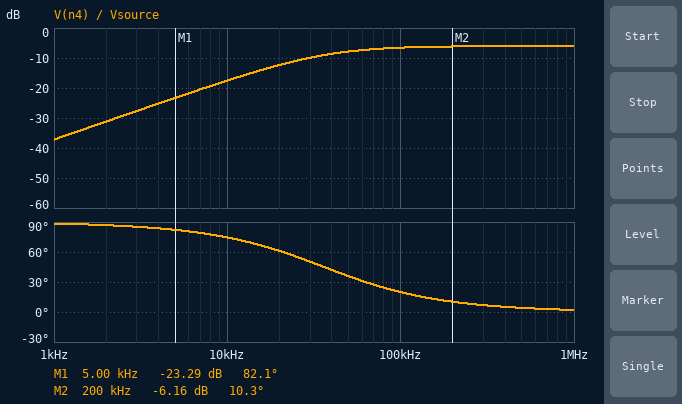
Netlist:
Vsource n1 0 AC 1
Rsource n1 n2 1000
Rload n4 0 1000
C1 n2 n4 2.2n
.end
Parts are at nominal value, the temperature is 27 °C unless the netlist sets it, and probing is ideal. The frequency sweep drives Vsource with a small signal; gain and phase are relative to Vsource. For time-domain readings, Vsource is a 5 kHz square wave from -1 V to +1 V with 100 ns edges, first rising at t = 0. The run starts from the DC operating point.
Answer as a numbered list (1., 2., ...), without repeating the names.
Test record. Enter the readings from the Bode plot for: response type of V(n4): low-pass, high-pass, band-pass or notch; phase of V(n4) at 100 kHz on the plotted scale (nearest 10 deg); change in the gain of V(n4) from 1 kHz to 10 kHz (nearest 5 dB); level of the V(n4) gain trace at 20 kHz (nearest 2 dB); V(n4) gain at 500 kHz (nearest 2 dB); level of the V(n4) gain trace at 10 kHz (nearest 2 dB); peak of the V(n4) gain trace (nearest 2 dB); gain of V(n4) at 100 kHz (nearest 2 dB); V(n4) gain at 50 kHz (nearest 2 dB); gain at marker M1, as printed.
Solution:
1. high-pass
2. 20 deg
3. 20 dB
4. -12 dB
5. -6 dB
6. -18 dB
7. -6 dB
8. -6 dB
9. -8 dB
10. -23.29 dB
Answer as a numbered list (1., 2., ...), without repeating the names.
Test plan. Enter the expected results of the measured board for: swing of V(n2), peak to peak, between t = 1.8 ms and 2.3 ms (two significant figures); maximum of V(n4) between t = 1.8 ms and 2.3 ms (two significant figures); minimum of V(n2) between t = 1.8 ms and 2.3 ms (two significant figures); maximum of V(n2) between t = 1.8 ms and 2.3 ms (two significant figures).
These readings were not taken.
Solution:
1. 2.0 V
2. 990 mV
3. -1.0 V
4. 1.0 V
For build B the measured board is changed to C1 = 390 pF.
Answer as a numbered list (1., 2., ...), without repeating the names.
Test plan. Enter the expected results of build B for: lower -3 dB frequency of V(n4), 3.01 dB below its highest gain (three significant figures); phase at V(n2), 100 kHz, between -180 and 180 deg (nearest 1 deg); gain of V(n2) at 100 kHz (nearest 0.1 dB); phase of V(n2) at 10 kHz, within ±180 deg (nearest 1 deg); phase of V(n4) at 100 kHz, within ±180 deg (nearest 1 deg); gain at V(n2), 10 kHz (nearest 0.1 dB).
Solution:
1. 204 kHz
2. -12 deg
3. -0.7 dB
4. -1 deg
5. 64 deg
6. 0 dB
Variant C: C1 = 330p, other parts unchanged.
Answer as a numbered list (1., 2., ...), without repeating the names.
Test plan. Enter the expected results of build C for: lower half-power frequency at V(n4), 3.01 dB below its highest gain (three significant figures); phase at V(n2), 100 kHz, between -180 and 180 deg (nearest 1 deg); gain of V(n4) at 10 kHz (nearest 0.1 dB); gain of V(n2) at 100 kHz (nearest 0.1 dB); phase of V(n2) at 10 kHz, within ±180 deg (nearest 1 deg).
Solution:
1. 241 kHz
2. -11 deg
3. -33.7 dB
4. -0.5 dB
5. -1 deg
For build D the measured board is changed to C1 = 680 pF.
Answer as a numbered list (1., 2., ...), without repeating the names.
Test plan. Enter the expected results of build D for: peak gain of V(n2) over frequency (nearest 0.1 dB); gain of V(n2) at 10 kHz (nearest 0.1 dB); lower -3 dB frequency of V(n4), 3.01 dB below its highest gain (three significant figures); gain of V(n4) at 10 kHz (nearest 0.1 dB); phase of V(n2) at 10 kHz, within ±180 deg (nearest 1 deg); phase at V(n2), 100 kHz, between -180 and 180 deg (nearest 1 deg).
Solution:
1. 0 dB
2. 0 dB
3. 117 kHz
4. -27.4 dB
5. -2 deg
6. -17 deg
